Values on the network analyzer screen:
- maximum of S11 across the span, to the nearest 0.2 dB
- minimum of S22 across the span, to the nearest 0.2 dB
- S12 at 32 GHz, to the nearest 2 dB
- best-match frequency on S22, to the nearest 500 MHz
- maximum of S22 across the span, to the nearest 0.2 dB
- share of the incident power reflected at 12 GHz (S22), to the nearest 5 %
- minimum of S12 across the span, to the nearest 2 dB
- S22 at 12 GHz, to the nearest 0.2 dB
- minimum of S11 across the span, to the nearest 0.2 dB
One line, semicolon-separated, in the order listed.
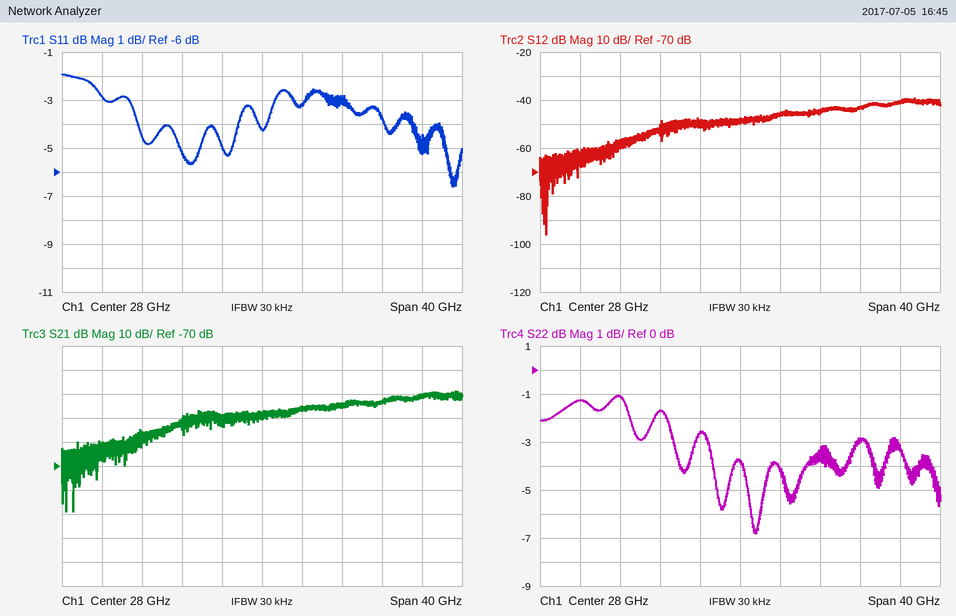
-2.0 dB; -6.8 dB; -46 dB; 29.5 GHz; -1.0 dB; 75 %; -96 dB; -1.2 dB; -6.6 dB
